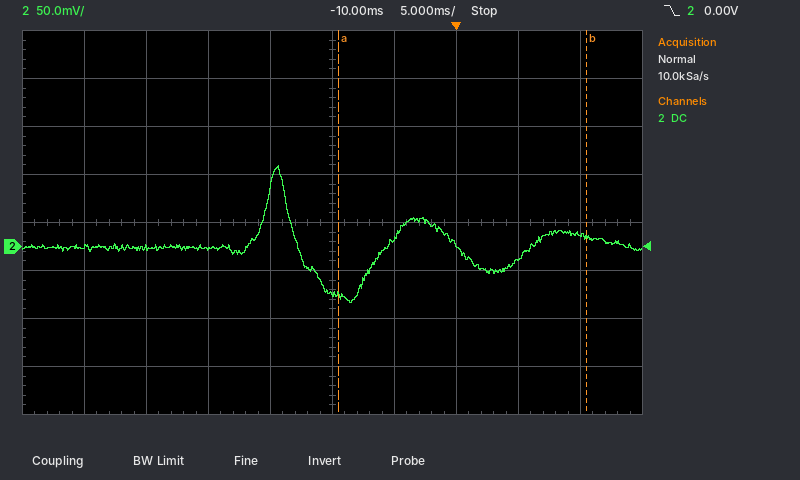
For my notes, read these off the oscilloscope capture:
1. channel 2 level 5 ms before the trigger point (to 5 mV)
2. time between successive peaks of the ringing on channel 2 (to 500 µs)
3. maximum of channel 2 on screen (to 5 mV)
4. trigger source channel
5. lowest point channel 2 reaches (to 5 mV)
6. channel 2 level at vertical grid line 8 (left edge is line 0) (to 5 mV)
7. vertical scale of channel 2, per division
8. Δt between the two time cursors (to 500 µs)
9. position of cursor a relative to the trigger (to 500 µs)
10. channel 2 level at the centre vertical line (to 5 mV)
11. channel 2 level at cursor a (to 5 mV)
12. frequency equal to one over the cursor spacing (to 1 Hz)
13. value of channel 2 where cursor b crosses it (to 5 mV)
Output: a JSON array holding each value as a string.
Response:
["10 mV", "11.5 ms", "85 mV", "channel 2", "-60 mV", "-15 mV", "50 mV", "20.0 ms", "-9.5 ms", "-50 mV", "-50 mV", "50 Hz", "10 mV"]
